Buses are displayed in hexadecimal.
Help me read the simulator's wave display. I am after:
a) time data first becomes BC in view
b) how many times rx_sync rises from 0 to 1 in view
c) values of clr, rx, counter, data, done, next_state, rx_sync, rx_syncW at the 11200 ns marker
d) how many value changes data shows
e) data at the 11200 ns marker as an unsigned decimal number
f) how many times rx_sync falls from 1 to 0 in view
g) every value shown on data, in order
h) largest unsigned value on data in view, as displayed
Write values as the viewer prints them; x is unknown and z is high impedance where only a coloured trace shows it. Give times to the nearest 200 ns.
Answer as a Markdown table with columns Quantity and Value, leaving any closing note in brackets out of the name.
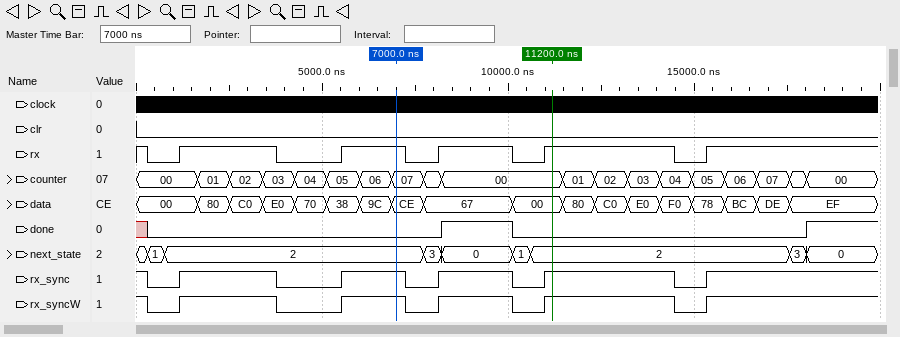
| Quantity | Value |
|---|---|
| time data first becomes BC in view | 15800 ns |
| how many times rx_sync rises from 0 to 1 in view | 5 |
| values of clr, rx, counter, data, done, next_state, rx_sync, rx_syncW at the 11200 ns marker | clr=0, rx=1, counter=00, data=00, done=0, next_state=2, rx_sync=1, rx_syncW=1 |
| how many value changes data shows | 17 |
| data at the 11200 ns marker as an unsigned decimal number | 0 |
| how many times rx_sync falls from 1 to 0 in view | 5 |
| every value shown on data, in order | 00, 80, C0, E0, 70, 38, 9C, CE, 67, 00, 80, C0, E0, F0, 78, BC, DE, EF |
| largest unsigned value on data in view, as displayed | F0 |
